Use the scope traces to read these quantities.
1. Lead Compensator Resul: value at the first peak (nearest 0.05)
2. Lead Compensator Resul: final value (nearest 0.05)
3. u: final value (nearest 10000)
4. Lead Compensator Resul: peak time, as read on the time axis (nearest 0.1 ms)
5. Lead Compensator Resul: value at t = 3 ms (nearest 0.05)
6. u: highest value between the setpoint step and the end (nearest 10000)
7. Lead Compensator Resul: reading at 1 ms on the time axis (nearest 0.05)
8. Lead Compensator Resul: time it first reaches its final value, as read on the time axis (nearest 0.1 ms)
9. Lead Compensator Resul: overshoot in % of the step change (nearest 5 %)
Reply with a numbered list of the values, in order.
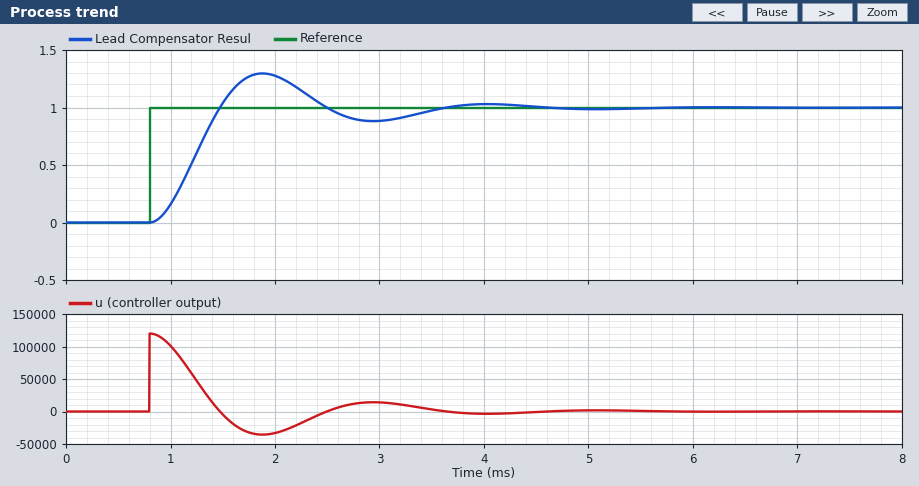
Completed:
1. 1.30
2. 1.00
3. 0
4. 1.9 ms
5. 0.90
6. 120000
7. 0.15
8. 1.5 ms
9. 30 %
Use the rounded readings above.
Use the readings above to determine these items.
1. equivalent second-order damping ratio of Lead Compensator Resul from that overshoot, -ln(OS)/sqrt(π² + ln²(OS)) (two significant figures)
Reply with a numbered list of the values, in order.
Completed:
1. 0.36
